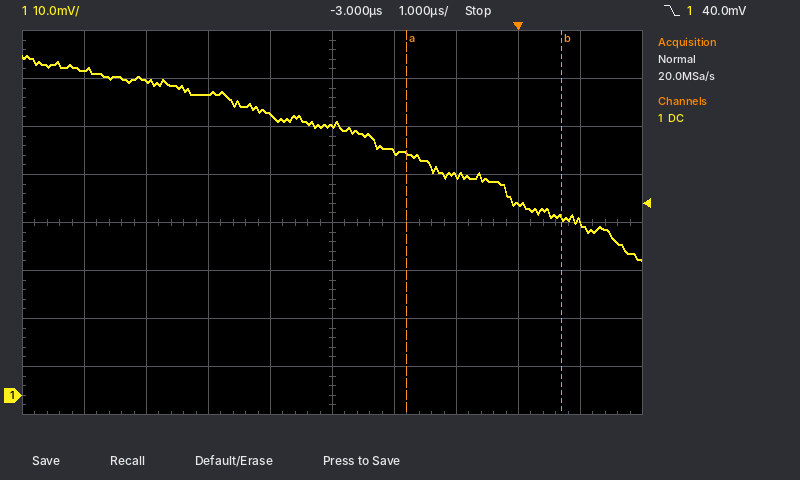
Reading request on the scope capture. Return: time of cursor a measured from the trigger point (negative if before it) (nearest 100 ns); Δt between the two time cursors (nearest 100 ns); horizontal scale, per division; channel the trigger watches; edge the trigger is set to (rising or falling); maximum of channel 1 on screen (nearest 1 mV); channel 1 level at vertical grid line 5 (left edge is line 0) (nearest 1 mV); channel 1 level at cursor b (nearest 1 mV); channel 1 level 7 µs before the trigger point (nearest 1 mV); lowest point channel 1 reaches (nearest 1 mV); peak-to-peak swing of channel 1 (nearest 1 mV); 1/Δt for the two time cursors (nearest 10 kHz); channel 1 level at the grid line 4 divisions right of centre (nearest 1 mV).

-1.8 µs
2.5 µs
1 µs
channel 1
falling
71 mV
56 mV
37 mV
68 mV
28 mV
43 mV
400 kHz
36 mV
